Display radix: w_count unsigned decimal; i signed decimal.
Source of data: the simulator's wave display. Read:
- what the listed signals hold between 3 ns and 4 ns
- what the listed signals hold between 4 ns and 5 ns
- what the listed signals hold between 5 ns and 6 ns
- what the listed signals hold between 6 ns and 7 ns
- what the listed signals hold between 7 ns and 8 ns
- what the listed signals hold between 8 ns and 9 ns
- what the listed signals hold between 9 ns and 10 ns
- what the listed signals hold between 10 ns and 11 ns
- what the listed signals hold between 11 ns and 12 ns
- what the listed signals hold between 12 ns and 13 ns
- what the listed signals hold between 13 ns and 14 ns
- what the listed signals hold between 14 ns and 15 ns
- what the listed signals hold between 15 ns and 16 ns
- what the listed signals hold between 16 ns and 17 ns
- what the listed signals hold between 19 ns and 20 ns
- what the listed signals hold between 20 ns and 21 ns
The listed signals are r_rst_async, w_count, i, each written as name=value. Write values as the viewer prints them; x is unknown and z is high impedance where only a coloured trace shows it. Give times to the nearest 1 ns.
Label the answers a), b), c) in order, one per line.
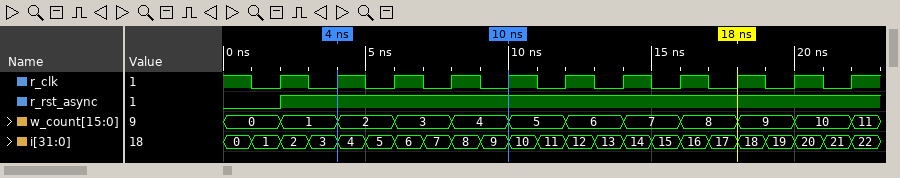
a) r_rst_async=1, w_count=1, i=3
b) r_rst_async=1, w_count=2, i=4
c) r_rst_async=1, w_count=2, i=5
d) r_rst_async=1, w_count=3, i=6
e) r_rst_async=1, w_count=3, i=7
f) r_rst_async=1, w_count=4, i=8
g) r_rst_async=1, w_count=4, i=9
h) r_rst_async=1, w_count=5, i=10
i) r_rst_async=1, w_count=5, i=11
j) r_rst_async=1, w_count=6, i=12
k) r_rst_async=1, w_count=6, i=13
l) r_rst_async=1, w_count=7, i=14
m) r_rst_async=1, w_count=7, i=15
n) r_rst_async=1, w_count=8, i=16
o) r_rst_async=1, w_count=9, i=19
p) r_rst_async=1, w_count=10, i=20
